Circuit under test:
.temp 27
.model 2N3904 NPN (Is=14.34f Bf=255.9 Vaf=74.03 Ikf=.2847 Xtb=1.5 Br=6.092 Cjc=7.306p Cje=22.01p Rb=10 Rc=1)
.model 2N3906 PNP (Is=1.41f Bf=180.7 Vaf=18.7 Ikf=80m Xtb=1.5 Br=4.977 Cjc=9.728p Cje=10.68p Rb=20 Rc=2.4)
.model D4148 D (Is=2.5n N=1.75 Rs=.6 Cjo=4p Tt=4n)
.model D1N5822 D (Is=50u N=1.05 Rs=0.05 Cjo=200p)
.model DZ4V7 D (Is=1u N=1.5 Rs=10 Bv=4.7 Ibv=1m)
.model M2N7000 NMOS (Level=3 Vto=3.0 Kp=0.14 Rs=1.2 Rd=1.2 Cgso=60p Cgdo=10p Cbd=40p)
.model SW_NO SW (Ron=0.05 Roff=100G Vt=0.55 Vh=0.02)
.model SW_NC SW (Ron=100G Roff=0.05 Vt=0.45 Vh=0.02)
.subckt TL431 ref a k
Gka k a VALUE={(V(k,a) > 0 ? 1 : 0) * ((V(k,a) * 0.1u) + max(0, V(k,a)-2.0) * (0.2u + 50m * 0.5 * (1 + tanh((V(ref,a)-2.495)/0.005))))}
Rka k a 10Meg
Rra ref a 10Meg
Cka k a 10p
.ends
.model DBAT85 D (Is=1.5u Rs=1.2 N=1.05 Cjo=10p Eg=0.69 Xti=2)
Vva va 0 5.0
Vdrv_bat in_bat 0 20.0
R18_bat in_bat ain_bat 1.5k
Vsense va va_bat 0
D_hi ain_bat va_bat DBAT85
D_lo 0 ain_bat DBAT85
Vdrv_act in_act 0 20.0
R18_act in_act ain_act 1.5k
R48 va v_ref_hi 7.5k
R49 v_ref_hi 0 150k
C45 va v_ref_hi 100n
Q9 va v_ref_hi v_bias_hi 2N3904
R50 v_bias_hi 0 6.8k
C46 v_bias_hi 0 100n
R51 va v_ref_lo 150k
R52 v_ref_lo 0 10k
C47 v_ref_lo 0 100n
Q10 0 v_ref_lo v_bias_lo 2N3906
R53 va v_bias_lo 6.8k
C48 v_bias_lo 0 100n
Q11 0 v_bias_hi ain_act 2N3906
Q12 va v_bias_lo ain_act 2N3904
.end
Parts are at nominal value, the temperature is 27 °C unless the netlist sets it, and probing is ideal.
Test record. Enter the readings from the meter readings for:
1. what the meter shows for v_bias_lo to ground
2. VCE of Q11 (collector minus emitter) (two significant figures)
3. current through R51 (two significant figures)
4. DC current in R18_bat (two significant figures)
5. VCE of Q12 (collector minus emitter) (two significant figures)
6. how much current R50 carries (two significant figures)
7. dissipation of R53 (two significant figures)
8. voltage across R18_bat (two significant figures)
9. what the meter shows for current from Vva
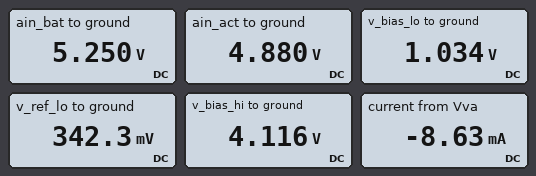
1.034 V
-4.9 V
31 µA
9.8 mA
120 mV
610 µA
2.3 mW
15 V
-8.63 mA
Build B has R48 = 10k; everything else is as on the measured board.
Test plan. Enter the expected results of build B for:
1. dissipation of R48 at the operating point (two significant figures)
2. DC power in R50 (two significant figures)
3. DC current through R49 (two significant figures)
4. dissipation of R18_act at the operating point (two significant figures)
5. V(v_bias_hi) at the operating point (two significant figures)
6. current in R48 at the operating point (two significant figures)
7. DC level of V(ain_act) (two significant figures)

11 µW
2.4 mW
31 µA
150 mW
4.0 V
33 µA
4.8 V
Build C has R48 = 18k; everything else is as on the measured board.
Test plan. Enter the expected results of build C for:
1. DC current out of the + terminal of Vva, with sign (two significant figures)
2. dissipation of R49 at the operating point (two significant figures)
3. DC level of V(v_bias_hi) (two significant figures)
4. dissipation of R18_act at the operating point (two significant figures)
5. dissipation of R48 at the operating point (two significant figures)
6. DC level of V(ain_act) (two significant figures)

-8.7 mA
130 µW
3.8 V
160 mW
18 µW
4.6 V
